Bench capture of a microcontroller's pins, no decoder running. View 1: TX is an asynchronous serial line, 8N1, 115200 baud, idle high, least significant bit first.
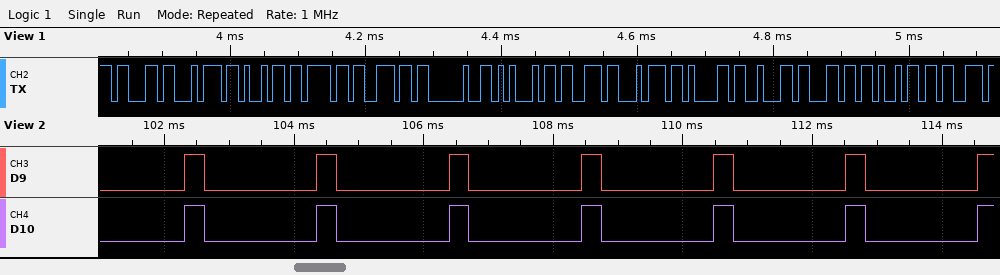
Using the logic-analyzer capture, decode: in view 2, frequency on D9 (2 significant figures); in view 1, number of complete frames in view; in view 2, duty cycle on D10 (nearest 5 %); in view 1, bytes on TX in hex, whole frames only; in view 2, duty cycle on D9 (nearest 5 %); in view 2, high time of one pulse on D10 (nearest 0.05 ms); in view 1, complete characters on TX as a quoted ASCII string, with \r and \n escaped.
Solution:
490 Hz
14
15 %
63 74 69 6F 6E 20 45 73 74 61 62 6C 69 73
15 %
0.30 ms
"ction Establis"
